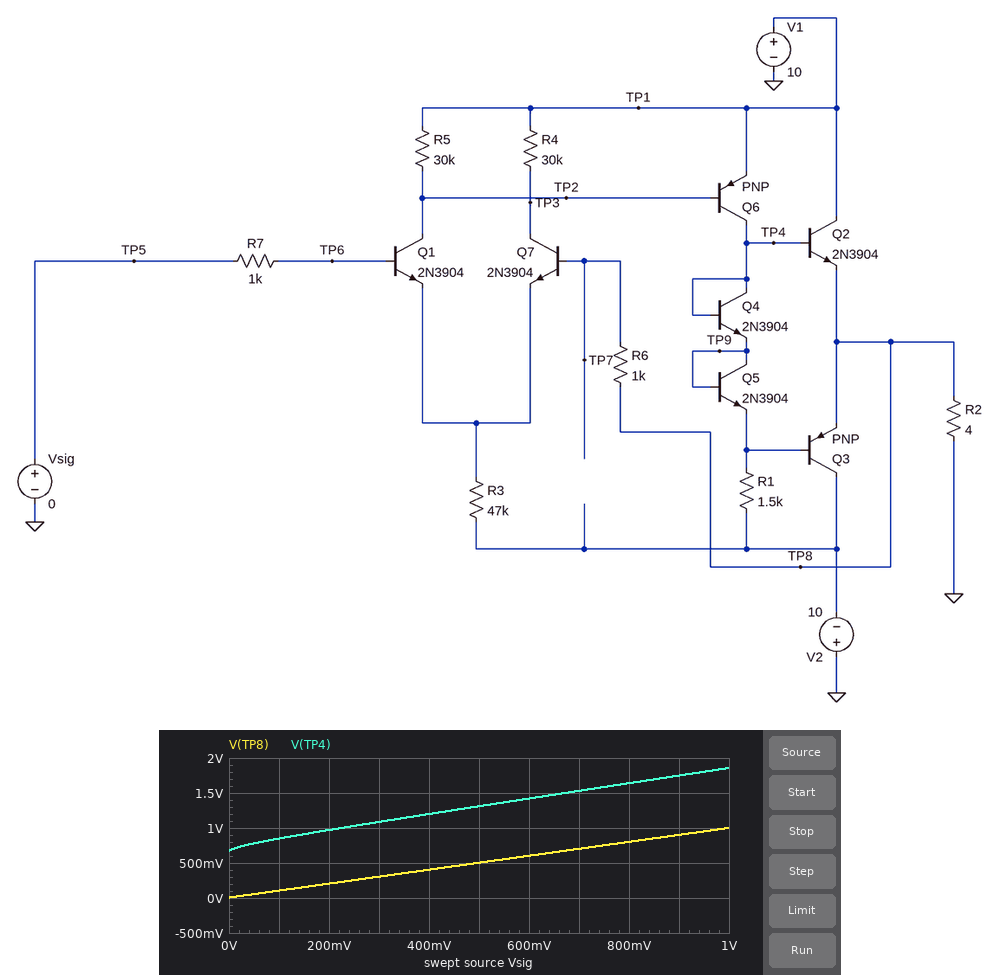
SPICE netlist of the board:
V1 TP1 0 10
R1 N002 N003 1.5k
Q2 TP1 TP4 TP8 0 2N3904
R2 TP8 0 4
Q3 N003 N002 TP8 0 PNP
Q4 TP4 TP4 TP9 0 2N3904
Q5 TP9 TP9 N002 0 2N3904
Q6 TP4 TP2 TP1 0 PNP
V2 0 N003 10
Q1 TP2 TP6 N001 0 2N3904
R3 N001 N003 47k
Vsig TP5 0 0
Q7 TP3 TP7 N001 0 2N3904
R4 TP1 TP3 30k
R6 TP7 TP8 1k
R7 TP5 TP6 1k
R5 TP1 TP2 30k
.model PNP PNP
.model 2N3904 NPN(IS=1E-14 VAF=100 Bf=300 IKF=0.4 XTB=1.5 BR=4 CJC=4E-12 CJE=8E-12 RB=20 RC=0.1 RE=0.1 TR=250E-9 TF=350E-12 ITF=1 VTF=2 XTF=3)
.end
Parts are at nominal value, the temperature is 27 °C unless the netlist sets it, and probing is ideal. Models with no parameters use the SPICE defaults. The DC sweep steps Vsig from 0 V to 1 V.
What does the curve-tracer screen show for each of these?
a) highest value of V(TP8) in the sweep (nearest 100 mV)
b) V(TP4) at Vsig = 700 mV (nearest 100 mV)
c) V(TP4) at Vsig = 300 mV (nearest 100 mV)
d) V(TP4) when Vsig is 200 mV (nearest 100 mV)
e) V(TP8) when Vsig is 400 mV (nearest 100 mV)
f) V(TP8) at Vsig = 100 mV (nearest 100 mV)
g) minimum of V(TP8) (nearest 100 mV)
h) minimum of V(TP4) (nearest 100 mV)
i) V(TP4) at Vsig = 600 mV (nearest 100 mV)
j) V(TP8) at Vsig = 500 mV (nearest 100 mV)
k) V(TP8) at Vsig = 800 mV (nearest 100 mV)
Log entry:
1.0 V
1.5 V
1.1 V
1.0 V
400 mV
100 mV
0 V
700 mV
1.4 V
500 mV
800 mV
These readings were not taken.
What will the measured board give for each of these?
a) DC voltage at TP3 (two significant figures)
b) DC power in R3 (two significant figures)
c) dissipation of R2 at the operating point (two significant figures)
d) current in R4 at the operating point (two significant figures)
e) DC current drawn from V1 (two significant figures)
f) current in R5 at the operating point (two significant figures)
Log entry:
6.7 V
1.9 mW
9.6 µW
110 µA
8.2 mA
27 µA
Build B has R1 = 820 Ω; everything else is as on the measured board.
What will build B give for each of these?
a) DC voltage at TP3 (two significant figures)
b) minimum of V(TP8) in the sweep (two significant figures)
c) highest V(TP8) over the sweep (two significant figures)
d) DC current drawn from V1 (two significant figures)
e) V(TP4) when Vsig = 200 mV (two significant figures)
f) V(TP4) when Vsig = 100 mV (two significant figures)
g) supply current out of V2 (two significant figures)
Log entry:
8.2 V
-22 mV
970 mV
12 mA
940 mV
810 mV
17 mA
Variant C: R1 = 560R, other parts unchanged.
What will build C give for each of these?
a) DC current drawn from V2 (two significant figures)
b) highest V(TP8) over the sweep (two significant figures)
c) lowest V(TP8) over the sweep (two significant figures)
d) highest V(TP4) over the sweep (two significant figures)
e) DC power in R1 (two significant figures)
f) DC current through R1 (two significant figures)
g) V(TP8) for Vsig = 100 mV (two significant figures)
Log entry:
35 mA
830 mV
-75 mV
1.7 V
150 mW
16 mA
16 mV
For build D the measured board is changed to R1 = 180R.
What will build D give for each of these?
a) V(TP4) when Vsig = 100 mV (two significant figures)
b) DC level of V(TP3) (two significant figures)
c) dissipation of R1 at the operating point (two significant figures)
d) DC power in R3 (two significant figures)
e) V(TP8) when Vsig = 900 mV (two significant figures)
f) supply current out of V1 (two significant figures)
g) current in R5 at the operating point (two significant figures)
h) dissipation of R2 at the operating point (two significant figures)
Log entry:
-3.6 V
10 V
130 mW
1.9 mW
-3.9 V
17 mA
28 µA
4.3 W
